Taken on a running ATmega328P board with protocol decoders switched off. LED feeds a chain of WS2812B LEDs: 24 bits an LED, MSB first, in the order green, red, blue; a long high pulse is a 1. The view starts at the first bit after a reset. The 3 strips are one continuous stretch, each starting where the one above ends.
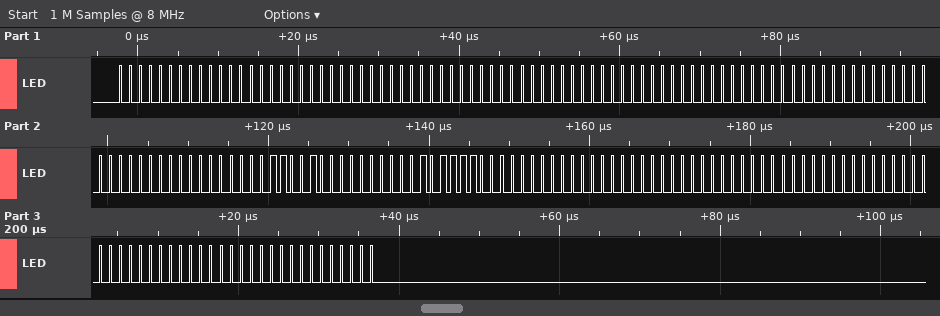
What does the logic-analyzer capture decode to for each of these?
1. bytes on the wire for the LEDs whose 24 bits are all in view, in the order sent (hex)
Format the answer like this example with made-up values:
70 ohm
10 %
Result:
00 00 00 00 00 00 00 00 00 00 00 00 32 00 5E 00 00 00 00 00 00 00 00 00
